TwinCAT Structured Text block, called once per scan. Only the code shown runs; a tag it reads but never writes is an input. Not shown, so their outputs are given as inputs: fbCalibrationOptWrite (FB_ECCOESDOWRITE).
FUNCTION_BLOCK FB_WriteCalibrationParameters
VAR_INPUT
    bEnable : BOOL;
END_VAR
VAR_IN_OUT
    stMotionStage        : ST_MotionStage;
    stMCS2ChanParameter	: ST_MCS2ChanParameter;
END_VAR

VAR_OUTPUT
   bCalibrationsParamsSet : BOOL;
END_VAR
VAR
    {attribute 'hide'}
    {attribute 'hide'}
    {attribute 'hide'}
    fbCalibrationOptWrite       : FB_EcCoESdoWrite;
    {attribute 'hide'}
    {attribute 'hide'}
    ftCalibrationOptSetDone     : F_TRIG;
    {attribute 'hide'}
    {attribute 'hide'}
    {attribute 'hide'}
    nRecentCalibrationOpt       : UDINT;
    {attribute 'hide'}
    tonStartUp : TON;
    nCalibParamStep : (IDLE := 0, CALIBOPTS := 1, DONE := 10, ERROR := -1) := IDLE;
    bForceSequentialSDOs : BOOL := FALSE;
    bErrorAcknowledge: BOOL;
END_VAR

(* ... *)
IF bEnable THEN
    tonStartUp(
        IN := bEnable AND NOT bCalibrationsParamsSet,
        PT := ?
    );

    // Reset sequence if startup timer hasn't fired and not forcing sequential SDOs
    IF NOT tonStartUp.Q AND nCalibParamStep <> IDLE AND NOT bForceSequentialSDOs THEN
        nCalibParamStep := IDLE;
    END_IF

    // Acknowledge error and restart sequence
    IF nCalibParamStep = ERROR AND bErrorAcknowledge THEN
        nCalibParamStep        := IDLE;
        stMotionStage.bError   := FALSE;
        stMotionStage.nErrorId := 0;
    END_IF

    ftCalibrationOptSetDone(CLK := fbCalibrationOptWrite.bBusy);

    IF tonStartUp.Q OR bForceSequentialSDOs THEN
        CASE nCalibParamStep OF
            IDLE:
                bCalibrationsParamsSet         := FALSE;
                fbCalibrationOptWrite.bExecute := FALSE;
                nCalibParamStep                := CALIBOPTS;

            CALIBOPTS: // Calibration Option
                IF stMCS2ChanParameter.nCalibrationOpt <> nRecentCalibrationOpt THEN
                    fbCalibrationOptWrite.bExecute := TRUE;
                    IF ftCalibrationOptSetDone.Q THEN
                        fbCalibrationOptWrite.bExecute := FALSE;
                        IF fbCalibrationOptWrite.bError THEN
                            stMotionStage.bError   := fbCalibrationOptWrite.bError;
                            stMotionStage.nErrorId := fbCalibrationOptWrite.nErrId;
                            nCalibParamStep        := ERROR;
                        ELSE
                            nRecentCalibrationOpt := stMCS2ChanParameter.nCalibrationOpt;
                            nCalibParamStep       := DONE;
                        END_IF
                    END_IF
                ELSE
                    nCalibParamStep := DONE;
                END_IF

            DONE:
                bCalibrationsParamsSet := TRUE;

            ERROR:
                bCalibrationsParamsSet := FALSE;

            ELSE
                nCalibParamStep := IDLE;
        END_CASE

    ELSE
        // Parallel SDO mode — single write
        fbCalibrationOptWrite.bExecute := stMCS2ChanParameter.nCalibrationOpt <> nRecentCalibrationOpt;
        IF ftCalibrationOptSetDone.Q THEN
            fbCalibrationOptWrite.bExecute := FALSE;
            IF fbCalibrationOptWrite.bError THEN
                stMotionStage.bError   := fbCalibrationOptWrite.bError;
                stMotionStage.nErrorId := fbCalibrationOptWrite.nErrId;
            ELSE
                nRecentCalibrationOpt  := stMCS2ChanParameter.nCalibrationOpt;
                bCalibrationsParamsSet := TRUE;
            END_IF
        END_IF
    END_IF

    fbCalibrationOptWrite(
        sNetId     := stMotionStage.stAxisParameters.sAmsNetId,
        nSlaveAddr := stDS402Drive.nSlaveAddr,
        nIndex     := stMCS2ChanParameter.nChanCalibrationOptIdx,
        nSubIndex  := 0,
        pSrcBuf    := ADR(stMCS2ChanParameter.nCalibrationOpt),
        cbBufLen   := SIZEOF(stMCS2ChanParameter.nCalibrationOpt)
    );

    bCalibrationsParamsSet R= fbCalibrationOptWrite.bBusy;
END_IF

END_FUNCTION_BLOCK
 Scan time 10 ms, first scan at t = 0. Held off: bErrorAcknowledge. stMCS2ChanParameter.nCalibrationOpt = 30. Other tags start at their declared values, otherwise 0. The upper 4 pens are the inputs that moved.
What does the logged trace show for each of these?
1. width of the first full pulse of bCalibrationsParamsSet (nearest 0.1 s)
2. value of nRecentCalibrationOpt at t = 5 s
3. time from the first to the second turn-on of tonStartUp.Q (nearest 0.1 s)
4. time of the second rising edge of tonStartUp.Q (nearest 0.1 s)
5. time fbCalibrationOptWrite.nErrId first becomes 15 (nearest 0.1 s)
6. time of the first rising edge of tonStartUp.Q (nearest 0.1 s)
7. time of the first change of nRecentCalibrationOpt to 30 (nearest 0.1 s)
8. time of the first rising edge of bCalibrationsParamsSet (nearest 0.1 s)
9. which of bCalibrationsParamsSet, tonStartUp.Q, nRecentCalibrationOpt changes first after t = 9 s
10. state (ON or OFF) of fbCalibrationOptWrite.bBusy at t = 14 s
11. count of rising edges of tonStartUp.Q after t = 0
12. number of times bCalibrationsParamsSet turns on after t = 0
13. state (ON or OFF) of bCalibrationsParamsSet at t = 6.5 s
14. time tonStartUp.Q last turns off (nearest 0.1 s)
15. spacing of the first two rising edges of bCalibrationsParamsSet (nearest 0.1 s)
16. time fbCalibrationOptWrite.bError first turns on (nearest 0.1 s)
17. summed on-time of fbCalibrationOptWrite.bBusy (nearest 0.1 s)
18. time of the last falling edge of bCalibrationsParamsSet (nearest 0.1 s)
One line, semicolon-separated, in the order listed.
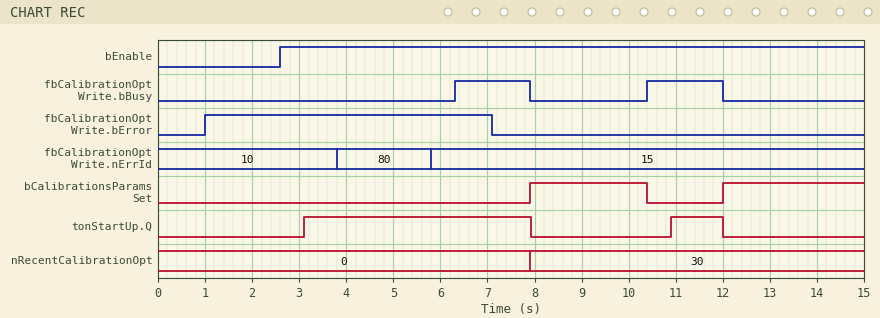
2.5 s; 0; 7.8 s; 10.9 s; 5.8 s; 3.1 s; 7.9 s; 7.9 s; bCalibrationsParamsSet; OFF; 2; 2; OFF; 12.0 s; 4.1 s; 1.0 s; 3.2 s; 10.4 s
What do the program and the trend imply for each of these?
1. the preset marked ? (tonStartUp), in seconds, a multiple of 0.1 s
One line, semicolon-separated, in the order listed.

0.5 s
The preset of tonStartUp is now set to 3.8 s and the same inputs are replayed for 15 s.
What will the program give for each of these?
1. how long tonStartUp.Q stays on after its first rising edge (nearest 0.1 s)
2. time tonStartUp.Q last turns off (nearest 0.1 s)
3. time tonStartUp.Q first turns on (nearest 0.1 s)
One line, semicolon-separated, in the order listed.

1.5 s; 7.9 s; 6.4 s
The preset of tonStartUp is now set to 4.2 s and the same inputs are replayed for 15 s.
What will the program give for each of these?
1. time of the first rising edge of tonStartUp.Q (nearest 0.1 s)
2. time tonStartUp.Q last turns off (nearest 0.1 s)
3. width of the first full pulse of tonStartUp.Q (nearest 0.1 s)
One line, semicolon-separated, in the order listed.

6.8 s; 7.9 s; 1.1 s
